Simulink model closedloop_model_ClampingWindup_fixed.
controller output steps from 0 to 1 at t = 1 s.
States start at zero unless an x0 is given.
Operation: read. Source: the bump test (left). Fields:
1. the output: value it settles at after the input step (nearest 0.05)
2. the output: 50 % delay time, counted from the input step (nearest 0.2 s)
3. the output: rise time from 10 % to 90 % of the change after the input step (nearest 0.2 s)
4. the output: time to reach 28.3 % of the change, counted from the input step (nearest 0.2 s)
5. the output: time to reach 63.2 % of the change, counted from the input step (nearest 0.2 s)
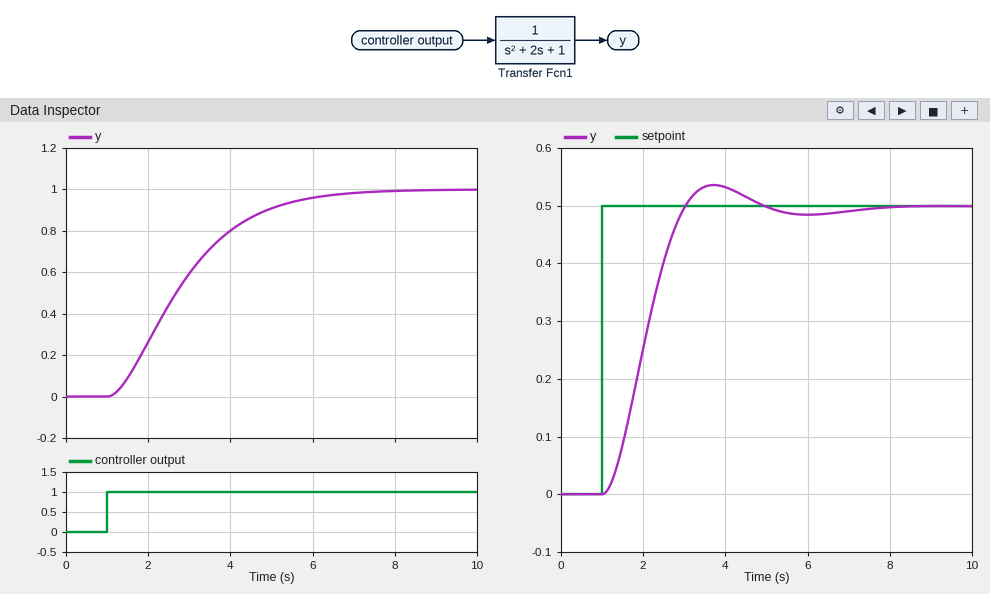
1.00
1.6 s
3.4 s
1.0 s
2.2 s
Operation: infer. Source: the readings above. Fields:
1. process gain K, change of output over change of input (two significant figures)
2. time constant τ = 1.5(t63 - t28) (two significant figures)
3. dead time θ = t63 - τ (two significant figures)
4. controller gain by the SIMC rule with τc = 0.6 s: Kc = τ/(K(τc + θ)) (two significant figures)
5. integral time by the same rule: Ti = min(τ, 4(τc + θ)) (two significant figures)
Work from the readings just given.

1.0
1.8 s
0.40 s
1.8
1.8 s
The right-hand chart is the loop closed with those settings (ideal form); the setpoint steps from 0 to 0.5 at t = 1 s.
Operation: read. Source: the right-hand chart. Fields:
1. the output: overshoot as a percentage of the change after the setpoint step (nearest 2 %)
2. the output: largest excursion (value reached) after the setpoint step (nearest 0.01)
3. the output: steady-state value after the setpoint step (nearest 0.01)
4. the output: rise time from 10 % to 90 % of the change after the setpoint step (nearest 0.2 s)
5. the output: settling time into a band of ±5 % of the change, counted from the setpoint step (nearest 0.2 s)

8 %
0.54
0.50
1.4 s
3.2 s
